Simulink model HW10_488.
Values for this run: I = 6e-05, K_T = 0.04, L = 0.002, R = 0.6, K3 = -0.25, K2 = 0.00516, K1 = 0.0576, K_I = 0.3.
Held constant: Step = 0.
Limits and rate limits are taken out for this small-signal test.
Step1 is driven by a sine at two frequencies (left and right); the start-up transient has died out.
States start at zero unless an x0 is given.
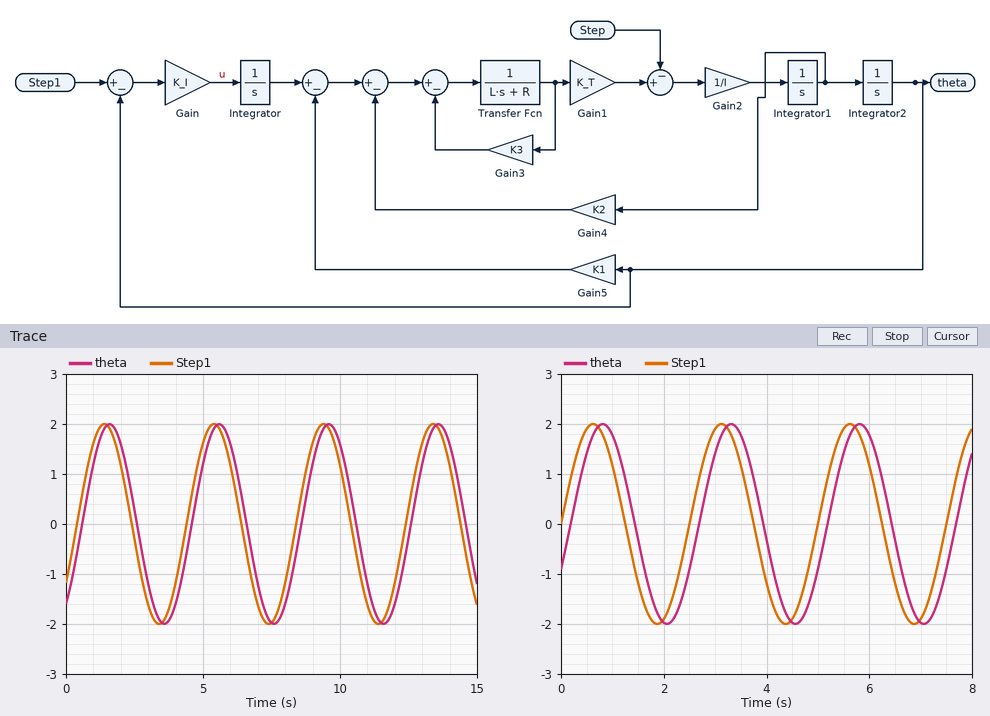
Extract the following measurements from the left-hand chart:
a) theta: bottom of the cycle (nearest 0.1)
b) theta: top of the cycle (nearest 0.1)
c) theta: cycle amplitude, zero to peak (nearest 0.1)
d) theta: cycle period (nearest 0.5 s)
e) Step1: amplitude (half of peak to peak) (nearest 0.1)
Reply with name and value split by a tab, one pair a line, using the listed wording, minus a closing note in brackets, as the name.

theta: bottom of the cycle	-2.0
theta: top of the cycle	2.0
theta: cycle amplitude, zero to peak	2.0
theta: cycle period	4.0 s
Step1: amplitude (half of peak to peak)	2.0
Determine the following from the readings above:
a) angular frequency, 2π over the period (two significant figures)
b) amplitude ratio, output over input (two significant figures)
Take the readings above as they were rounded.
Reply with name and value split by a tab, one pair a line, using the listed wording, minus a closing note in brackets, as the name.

angular frequency, 2π over the period	1.6 rad/s
amplitude ratio, output over input	1.0
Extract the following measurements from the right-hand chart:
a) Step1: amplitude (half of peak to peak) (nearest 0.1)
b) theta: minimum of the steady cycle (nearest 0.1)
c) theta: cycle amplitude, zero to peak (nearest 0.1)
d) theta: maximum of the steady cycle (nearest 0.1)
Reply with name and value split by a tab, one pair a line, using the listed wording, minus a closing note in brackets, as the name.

Step1: amplitude (half of peak to peak)	2.0
theta: minimum of the steady cycle	-2.0
theta: cycle amplitude, zero to peak	2.0
theta: maximum of the steady cycle	2.0
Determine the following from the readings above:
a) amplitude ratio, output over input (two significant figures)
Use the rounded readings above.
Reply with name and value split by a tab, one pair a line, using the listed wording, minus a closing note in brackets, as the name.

amplitude ratio, output over input	1.0
